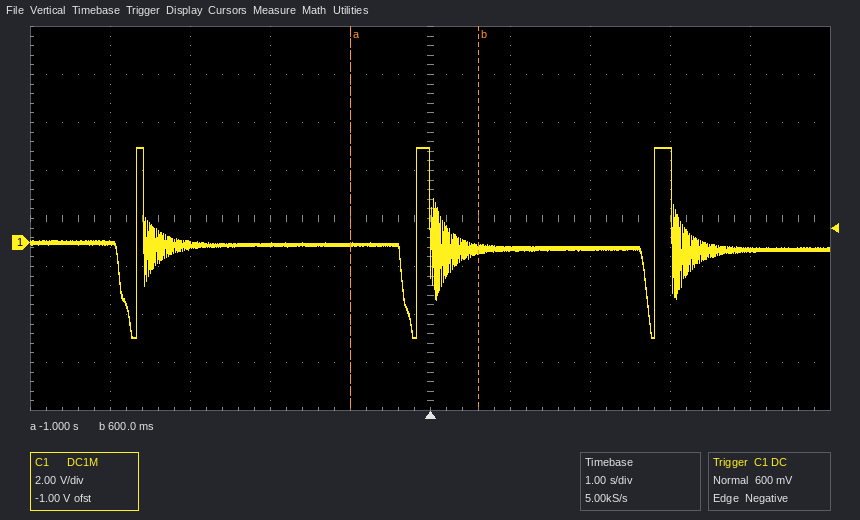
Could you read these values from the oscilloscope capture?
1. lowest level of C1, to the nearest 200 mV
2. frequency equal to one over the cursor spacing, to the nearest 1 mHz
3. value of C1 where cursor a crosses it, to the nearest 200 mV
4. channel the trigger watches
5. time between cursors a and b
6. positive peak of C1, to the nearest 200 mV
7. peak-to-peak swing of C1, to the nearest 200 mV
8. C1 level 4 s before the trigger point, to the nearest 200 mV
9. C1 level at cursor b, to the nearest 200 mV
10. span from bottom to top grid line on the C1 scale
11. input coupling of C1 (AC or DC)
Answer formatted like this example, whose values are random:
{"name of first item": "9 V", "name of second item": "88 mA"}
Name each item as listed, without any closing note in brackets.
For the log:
{"lowest level of C1, to the nearest 200 mV": "-4.0 V", "frequency equal to one over the cursor spacing, to the nearest 1 mHz": "625 mHz", "value of C1 where cursor a crosses it, to the nearest 200 mV": "0.0 V", "channel the trigger watches": "C1", "time between cursors a and b": "1.6 s", "positive peak of C1, to the nearest 200 mV": "4.0 V", "peak-to-peak swing of C1, to the nearest 200 mV": "8.0 V", "C1 level 4 s before the trigger point, to the nearest 200 mV": "0.0 V", "C1 level at cursor b, to the nearest 200 mV": "-200 mV", "span from bottom to top grid line on the C1 scale": "16 V", "input coupling of C1": "DC"}
